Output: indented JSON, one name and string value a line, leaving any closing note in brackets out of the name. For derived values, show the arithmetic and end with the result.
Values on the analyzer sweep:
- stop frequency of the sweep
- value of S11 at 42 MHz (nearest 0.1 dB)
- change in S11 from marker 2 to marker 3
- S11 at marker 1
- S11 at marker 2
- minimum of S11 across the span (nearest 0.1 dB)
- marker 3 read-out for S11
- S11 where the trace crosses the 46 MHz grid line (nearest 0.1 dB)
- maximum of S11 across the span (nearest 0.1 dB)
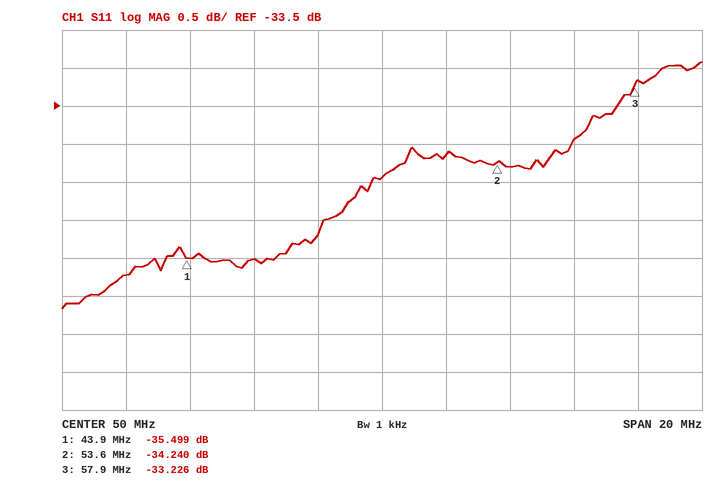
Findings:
{
  "stop frequency of the sweep": "60 MHz",
  "value of S11 at 42 MHz": "-35.7 dB",
  "change in S11 from marker 2 to marker 3": "-33.226 − (-34.24) = 1.014 dB",
  "S11 at marker 1": "-35.499 dB",
  "S11 at marker 2": "-34.240 dB",
  "minimum of S11 across the span": "-36.2 dB",
  "marker 3 read-out for S11": "-33.226 dB",
  "S11 where the trace crosses the 46 MHz grid line": "-35.5 dB",
  "maximum of S11 across the span": "-32.9 dB"
}
